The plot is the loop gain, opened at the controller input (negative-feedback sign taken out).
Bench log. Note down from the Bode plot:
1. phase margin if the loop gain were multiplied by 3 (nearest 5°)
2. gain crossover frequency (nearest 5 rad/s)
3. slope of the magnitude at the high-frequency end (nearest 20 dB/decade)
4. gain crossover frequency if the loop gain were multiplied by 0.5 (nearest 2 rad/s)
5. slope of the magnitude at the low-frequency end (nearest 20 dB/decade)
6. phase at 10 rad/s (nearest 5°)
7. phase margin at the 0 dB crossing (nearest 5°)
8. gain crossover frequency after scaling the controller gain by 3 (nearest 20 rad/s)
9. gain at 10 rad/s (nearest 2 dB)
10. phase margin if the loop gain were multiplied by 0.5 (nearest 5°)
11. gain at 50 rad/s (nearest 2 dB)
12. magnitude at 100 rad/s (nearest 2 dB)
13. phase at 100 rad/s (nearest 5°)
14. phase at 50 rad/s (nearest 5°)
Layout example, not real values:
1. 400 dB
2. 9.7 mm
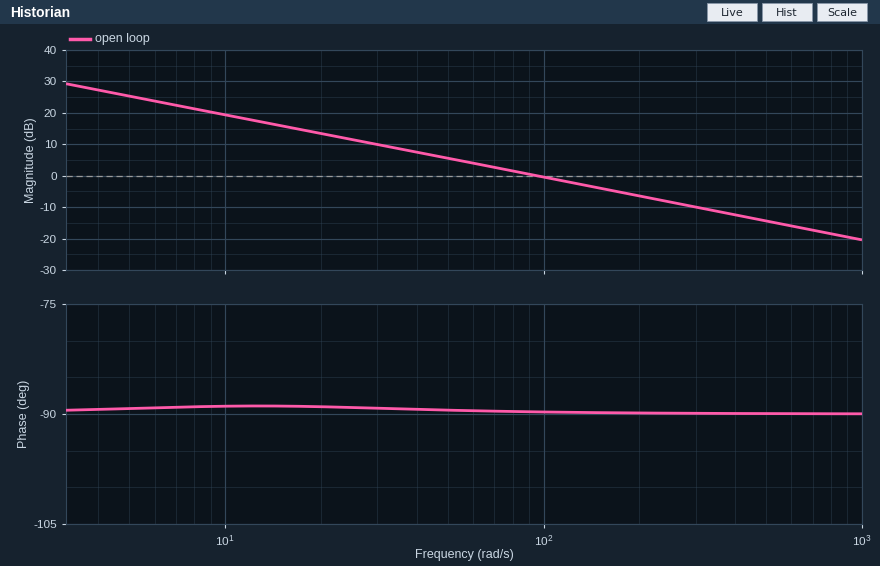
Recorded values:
1. 90°
2. 95 rad/s
3. -20 dB/decade
4. 48 rad/s
5. -20 dB/decade
6. -90°
7. 90°
8. 280 rad/s
9. 20 dB
10. 90°
11. 6 dB
12. 0 dB
13. -90°
14. -90°
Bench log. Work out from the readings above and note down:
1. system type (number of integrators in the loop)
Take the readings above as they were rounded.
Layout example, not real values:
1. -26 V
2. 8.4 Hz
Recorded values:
1. 1
